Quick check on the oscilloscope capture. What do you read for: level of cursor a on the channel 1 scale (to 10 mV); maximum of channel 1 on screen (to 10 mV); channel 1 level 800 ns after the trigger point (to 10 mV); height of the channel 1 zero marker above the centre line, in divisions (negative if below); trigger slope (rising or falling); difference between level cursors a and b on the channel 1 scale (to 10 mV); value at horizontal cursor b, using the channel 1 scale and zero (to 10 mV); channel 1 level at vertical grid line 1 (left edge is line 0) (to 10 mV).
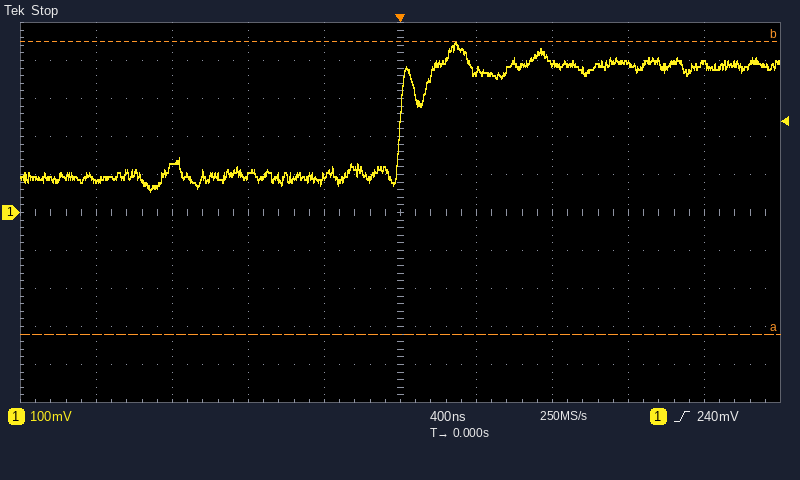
-320 mV
450 mV
390 mV
0.0 div
rising
770 mV
450 mV
90 mV
